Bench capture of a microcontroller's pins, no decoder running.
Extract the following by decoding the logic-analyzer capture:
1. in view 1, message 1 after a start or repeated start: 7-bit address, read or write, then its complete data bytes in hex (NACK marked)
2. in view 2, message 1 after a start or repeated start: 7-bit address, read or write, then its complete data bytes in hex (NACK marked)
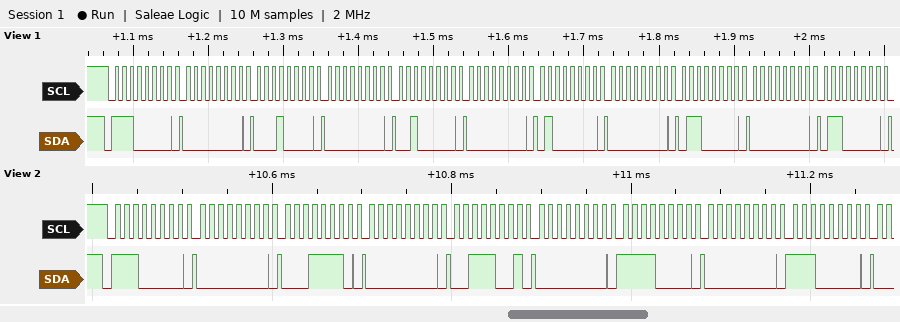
0x70 write: 00 10 00 20 00 40 00 60 00 60
0x70 write: 00 1E 00 39 00 F0 00 E0
